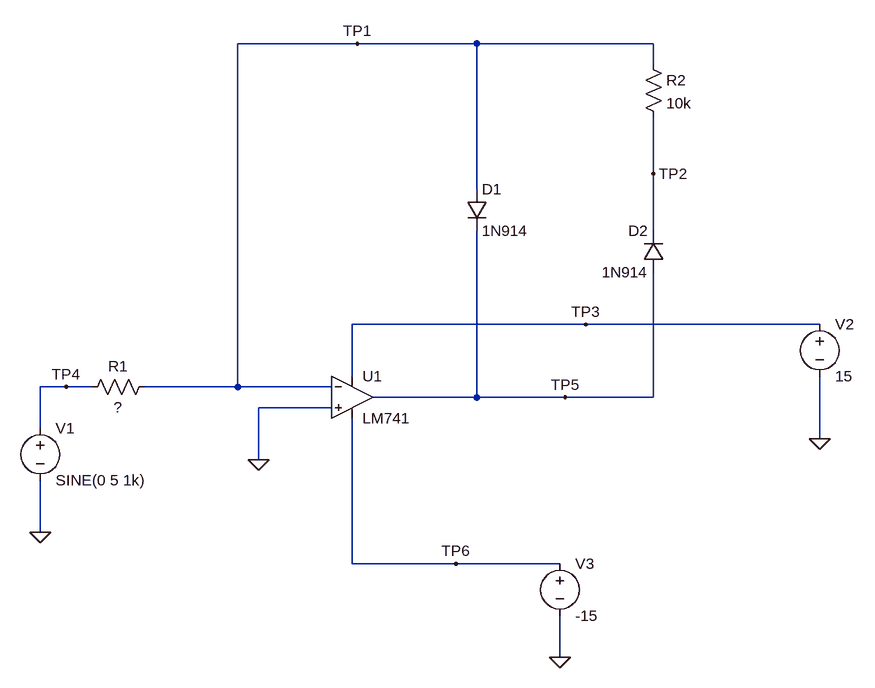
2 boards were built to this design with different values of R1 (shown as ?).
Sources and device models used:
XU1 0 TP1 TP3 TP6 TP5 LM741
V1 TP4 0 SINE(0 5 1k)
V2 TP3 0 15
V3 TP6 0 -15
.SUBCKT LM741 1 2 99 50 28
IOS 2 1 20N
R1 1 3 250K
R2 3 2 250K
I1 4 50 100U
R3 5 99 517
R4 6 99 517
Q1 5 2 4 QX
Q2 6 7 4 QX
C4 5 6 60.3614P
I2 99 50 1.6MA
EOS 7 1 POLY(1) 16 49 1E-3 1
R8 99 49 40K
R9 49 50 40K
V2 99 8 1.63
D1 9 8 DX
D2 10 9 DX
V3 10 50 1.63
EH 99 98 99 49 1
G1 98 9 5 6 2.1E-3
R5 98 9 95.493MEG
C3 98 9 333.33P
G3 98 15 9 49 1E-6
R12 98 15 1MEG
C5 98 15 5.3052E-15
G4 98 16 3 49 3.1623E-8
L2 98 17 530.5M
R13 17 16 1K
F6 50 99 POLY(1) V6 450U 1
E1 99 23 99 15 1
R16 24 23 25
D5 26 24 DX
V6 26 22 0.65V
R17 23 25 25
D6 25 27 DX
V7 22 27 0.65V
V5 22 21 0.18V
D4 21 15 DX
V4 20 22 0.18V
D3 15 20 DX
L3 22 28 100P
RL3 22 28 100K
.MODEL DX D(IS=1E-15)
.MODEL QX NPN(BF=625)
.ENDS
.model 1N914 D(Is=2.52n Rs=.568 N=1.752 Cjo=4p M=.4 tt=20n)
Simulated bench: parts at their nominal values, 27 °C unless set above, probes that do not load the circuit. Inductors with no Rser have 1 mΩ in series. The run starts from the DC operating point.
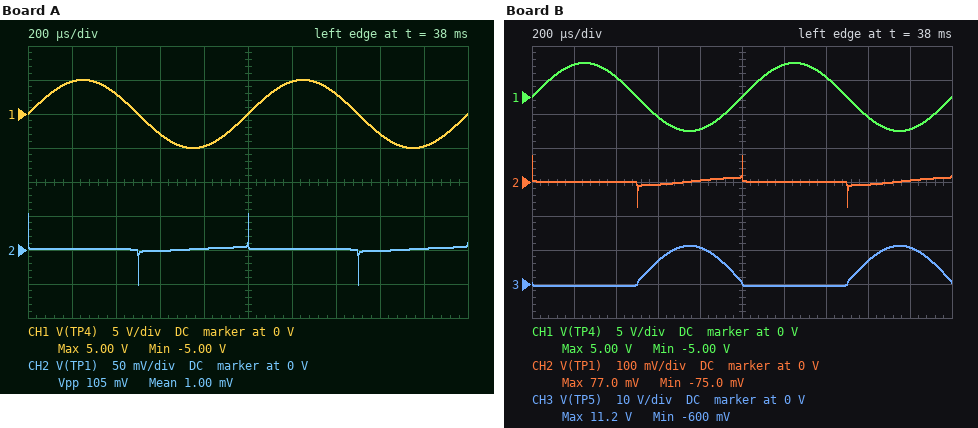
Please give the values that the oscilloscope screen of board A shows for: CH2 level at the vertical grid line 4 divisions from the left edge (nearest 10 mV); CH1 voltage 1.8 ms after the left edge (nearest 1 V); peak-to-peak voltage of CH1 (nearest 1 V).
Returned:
0 V
-5 V
10 V
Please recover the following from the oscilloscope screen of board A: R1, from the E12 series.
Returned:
18 kΩ
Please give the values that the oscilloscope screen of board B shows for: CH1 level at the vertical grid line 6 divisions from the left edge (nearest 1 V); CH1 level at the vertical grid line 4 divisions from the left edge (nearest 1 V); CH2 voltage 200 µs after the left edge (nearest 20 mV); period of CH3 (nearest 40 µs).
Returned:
5 V
-5 V
0 V
1.00 ms
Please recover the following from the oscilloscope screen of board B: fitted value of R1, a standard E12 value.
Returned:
4.7 kΩ
